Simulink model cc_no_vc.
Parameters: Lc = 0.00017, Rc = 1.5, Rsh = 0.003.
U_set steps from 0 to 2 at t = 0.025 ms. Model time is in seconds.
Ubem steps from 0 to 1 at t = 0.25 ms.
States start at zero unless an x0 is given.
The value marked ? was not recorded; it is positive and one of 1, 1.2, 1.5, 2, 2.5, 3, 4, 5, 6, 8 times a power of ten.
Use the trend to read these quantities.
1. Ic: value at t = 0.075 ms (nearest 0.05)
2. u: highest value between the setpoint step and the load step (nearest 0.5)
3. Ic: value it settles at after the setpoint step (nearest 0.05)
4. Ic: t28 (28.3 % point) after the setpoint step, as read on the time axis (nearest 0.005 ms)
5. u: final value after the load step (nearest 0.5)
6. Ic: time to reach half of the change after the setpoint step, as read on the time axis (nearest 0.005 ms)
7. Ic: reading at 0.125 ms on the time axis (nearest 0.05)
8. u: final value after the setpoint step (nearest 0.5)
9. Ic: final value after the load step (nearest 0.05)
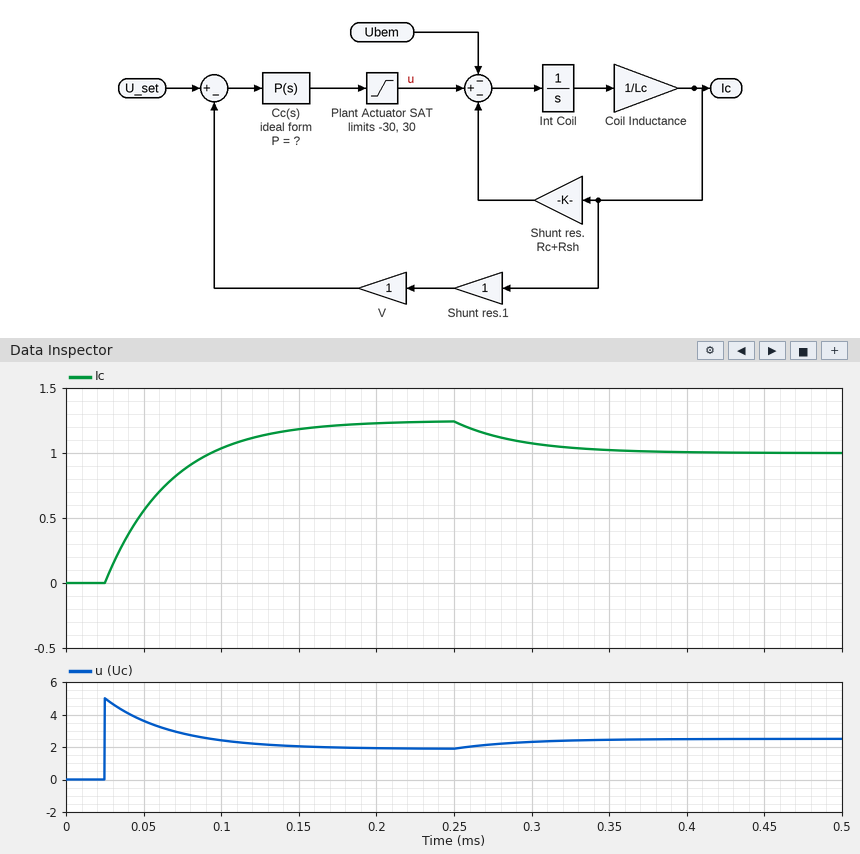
0.85
5.0
1.25
0.040 ms
2.5
0.055 ms
1.15
2.0
1.00
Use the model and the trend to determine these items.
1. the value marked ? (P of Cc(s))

2.5
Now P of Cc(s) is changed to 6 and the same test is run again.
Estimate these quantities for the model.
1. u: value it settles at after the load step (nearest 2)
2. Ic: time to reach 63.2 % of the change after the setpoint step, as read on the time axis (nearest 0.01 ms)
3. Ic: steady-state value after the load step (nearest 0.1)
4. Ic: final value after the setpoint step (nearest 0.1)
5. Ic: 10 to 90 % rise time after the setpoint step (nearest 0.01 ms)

4
0.05 ms
1.5
1.6
0.05 ms
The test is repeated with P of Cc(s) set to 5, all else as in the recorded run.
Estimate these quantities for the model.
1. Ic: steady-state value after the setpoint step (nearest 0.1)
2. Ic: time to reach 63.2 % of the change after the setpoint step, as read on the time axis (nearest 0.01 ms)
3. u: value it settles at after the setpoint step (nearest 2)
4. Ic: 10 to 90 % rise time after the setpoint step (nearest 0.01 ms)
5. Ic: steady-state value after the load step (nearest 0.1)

1.5
0.05 ms
2
0.06 ms
1.4
